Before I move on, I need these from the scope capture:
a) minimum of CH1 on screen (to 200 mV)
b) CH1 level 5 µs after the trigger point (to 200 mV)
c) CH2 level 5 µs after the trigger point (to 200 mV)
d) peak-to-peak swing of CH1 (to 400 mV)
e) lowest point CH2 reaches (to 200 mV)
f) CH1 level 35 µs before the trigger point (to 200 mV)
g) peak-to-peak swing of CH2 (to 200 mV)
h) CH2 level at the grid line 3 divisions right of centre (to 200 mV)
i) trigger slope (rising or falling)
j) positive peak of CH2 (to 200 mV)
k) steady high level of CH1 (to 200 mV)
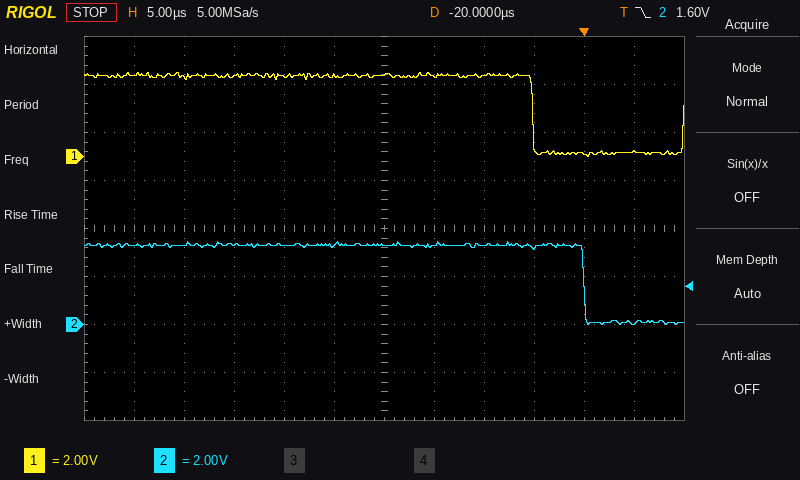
0.0 V
200 mV
0.0 V
3.6 V
0.0 V
3.4 V
3.4 V
3.2 V
falling
3.4 V
3.4 V
